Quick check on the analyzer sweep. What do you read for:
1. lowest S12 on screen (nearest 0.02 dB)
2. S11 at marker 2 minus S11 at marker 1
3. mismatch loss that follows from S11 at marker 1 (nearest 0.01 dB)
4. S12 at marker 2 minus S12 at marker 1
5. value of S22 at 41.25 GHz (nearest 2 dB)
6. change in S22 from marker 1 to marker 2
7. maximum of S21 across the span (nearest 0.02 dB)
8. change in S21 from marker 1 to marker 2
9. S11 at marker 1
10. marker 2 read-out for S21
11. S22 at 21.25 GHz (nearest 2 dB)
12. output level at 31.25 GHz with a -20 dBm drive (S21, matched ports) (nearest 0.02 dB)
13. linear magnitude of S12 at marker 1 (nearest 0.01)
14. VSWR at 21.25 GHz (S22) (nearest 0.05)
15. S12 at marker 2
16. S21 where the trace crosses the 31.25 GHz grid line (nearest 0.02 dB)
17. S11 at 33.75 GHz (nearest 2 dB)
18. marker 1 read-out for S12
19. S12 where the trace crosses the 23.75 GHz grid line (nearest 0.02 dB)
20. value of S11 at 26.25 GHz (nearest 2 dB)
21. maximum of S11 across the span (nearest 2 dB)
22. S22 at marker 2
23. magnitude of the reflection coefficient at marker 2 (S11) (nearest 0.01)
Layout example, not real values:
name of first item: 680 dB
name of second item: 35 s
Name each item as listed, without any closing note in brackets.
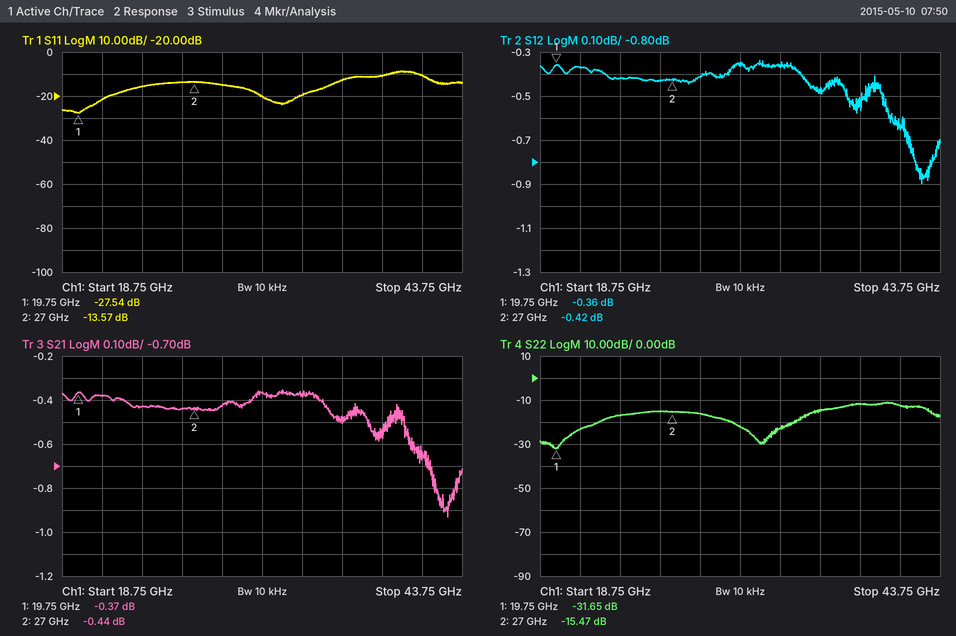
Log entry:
lowest S12 on screen: -0.90 dB
S11 at marker 2 minus S11 at marker 1: 13.97 dB
mismatch loss that follows from S11 at marker 1: 0.01 dB
S12 at marker 2 minus S12 at marker 1: -0.06 dB
value of S22 at 41.25 GHz: -12 dB
change in S22 from marker 1 to marker 2: 16.18 dB
maximum of S21 across the span: -0.36 dB
change in S21 from marker 1 to marker 2: -0.07 dB
S11 at marker 1: -27.54 dB
marker 2 read-out for S21: -0.44 dB
S22 at 21.25 GHz: -24 dB
output level at 31.25 GHz with a -20 dBm drive (S21, matched ports): -20.36 dBm
linear magnitude of S12 at marker 1: 0.96
VSWR at 21.25 GHz (S22): 1.15
S12 at marker 2: -0.42 dB
S21 where the trace crosses the 31.25 GHz grid line: -0.36 dB
S11 at 33.75 GHz: -20 dB
marker 1 read-out for S12: -0.36 dB
S12 where the trace crosses the 23.75 GHz grid line: -0.42 dB
value of S11 at 26.25 GHz: -14 dB
maximum of S11 across the span: -8 dB
S22 at marker 2: -15.47 dB
magnitude of the reflection coefficient at marker 2 (S11): 0.21
